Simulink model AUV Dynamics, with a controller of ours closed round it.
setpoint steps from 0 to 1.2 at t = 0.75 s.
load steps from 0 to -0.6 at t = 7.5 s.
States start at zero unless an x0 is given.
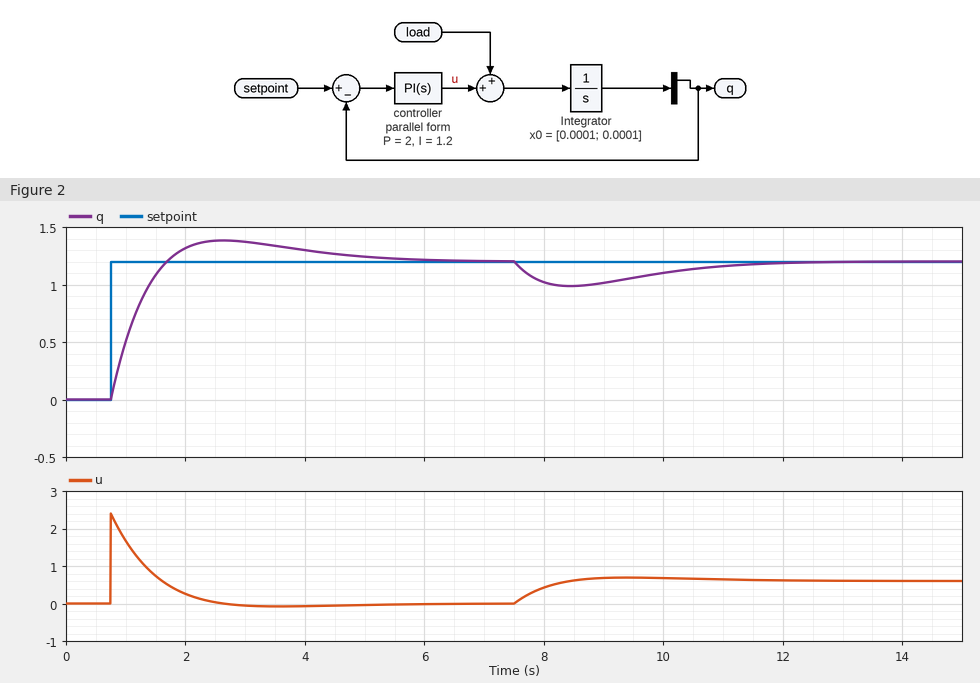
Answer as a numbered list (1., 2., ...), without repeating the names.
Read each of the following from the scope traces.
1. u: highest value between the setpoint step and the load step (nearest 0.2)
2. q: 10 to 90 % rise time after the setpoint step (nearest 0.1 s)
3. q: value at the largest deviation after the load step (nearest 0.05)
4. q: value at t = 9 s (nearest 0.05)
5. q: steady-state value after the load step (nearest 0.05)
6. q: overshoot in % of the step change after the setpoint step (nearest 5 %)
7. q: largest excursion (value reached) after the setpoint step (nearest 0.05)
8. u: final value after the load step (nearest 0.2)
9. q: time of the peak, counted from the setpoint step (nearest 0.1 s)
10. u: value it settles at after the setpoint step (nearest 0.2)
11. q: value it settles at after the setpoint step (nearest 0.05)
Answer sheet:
1. 2.4
2. 0.7 s
3. 1.00
4. 1.00
5. 1.20
6. 15 %
7. 1.40
8. 0.6
9. 1.9 s
10. 0.0
11. 1.20
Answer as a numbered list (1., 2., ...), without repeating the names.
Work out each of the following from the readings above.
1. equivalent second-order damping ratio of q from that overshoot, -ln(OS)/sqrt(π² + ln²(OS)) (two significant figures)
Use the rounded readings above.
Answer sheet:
1. 0.52
